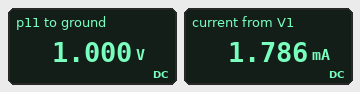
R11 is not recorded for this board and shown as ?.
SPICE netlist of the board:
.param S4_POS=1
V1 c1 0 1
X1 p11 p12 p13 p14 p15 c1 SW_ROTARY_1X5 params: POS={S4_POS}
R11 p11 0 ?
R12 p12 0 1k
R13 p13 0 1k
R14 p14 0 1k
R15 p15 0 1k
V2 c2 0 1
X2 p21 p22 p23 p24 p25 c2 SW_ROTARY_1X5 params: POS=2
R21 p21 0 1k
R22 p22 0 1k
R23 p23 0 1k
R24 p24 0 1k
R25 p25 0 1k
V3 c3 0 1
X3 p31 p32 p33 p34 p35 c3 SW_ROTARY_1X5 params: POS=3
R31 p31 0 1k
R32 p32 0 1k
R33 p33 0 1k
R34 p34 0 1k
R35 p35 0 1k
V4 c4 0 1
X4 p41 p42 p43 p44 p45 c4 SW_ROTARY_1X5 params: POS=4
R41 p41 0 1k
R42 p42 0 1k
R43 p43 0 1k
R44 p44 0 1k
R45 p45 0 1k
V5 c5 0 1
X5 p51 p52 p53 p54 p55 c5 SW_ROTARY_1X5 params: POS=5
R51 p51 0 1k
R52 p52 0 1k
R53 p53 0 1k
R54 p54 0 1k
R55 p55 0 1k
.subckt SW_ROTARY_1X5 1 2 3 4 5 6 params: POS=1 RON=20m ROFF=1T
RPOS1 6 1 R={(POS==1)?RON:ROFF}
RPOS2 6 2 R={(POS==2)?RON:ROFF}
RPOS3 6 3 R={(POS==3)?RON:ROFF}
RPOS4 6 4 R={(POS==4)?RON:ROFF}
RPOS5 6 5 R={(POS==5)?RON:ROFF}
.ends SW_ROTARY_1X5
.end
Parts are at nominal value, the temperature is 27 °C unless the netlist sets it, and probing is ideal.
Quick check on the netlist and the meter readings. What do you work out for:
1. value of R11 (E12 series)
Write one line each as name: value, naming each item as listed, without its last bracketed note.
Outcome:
value of R11: 560 Ω
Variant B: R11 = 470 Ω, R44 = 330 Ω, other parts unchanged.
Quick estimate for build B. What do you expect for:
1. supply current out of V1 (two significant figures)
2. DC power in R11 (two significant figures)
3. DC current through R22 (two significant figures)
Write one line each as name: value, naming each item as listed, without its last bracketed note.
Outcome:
supply current out of V1: 2.1 mA
DC power in R11: 2.1 mW
DC current through R22: 1.0 mA
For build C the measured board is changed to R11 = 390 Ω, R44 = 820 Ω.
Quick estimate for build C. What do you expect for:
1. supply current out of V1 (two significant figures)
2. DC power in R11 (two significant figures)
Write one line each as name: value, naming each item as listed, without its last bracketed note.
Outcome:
supply current out of V1: 2.6 mA
DC power in R11: 2.6 mW
